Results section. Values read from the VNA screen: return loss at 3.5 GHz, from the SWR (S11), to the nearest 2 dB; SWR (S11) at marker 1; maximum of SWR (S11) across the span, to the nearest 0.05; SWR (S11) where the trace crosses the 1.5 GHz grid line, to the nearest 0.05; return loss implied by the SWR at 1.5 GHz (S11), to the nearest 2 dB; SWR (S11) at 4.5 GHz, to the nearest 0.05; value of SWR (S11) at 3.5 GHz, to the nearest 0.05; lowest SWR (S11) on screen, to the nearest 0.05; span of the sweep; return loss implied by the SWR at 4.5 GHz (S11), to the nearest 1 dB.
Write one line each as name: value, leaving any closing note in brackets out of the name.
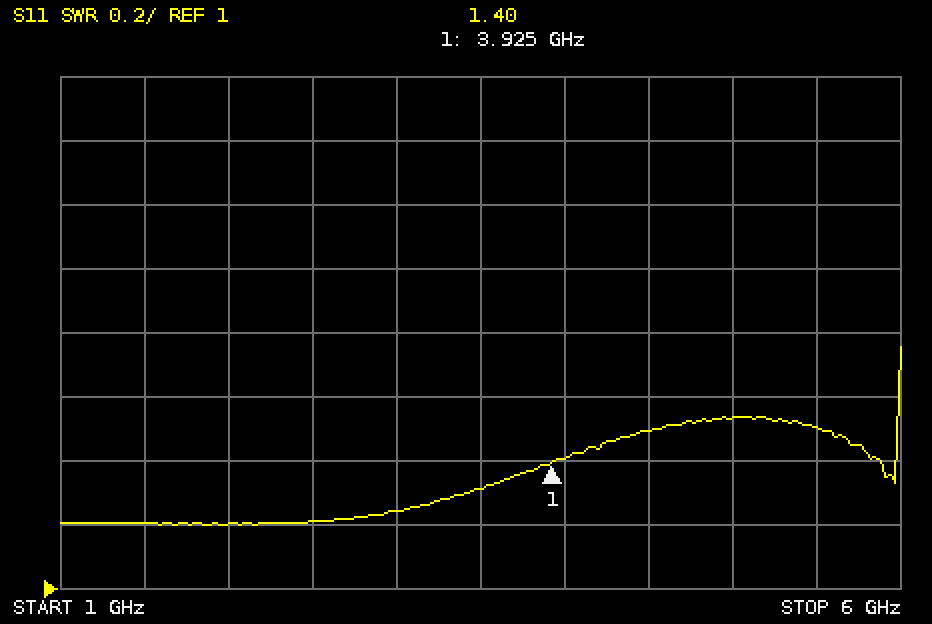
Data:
return loss at 3.5 GHz, from the SWR (S11), to the nearest 2 dB: 18 dB
SWR (S11) at marker 1: 1.40
maximum of SWR (S11) across the span, to the nearest 0.05: 1.75
SWR (S11) where the trace crosses the 1.5 GHz grid line, to the nearest 0.05: 1.20
return loss implied by the SWR at 1.5 GHz (S11), to the nearest 2 dB: 20 dB
SWR (S11) at 4.5 GHz, to the nearest 0.05: 1.50
value of SWR (S11) at 3.5 GHz, to the nearest 0.05: 1.30
lowest SWR (S11) on screen, to the nearest 0.05: 1.20
span of the sweep: 5 GHz
return loss implied by the SWR at 4.5 GHz (S11), to the nearest 1 dB: 14 dB
